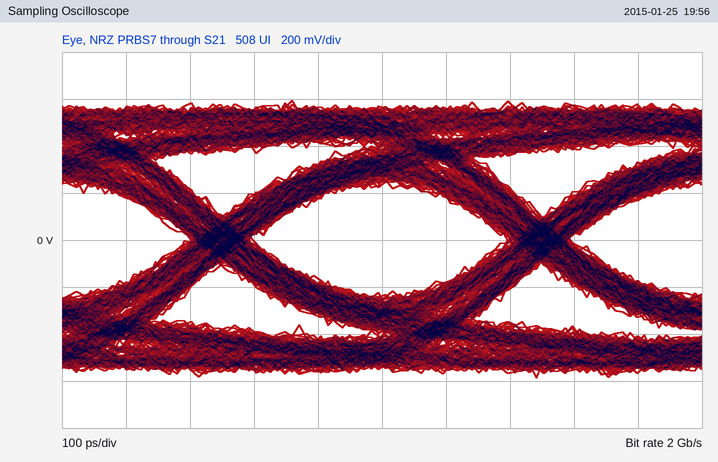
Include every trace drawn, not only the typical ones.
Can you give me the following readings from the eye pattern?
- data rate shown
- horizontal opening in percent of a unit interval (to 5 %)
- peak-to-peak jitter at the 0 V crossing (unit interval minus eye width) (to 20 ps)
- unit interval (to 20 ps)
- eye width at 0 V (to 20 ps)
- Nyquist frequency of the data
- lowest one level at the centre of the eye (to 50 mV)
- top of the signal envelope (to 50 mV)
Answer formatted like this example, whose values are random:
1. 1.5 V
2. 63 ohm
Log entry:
1. 2 Gb/s
2. 80 %
3. 100 ps
4. 500 ps
5. 400 ps
6. 1 GHz
7. 250 mV
8. 600 mV
